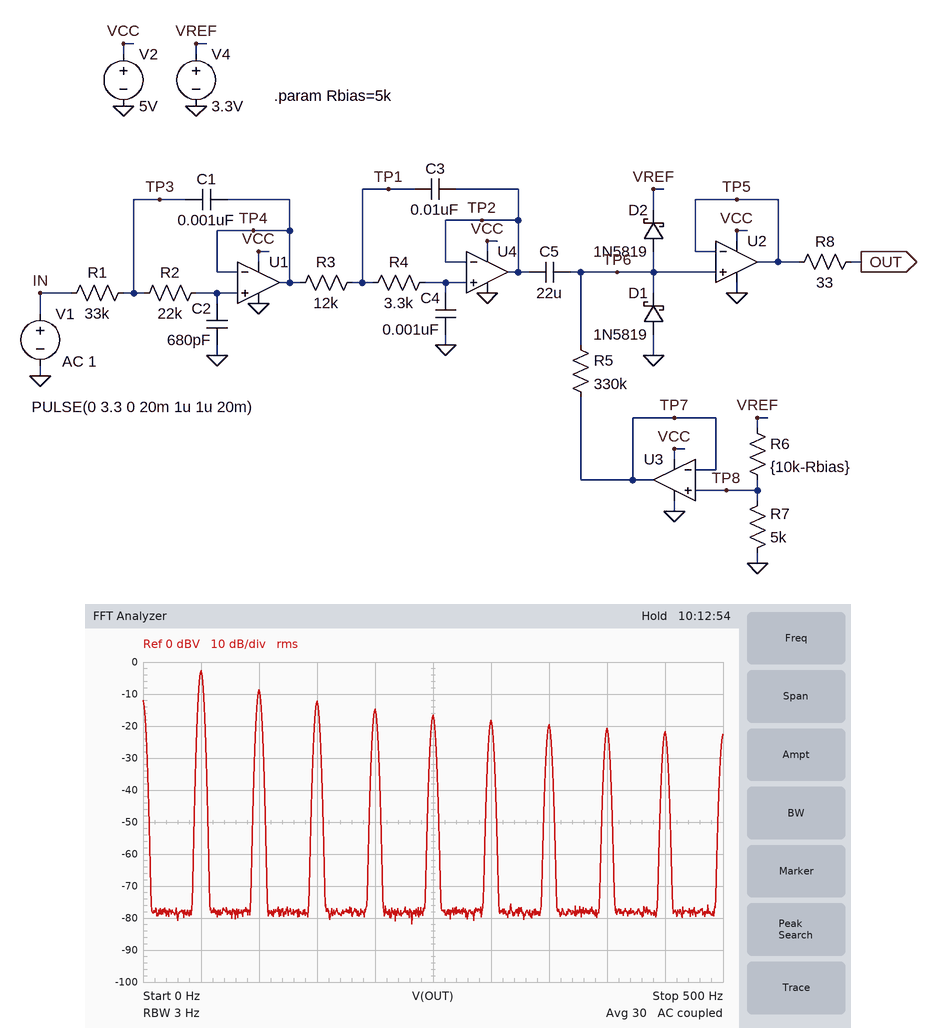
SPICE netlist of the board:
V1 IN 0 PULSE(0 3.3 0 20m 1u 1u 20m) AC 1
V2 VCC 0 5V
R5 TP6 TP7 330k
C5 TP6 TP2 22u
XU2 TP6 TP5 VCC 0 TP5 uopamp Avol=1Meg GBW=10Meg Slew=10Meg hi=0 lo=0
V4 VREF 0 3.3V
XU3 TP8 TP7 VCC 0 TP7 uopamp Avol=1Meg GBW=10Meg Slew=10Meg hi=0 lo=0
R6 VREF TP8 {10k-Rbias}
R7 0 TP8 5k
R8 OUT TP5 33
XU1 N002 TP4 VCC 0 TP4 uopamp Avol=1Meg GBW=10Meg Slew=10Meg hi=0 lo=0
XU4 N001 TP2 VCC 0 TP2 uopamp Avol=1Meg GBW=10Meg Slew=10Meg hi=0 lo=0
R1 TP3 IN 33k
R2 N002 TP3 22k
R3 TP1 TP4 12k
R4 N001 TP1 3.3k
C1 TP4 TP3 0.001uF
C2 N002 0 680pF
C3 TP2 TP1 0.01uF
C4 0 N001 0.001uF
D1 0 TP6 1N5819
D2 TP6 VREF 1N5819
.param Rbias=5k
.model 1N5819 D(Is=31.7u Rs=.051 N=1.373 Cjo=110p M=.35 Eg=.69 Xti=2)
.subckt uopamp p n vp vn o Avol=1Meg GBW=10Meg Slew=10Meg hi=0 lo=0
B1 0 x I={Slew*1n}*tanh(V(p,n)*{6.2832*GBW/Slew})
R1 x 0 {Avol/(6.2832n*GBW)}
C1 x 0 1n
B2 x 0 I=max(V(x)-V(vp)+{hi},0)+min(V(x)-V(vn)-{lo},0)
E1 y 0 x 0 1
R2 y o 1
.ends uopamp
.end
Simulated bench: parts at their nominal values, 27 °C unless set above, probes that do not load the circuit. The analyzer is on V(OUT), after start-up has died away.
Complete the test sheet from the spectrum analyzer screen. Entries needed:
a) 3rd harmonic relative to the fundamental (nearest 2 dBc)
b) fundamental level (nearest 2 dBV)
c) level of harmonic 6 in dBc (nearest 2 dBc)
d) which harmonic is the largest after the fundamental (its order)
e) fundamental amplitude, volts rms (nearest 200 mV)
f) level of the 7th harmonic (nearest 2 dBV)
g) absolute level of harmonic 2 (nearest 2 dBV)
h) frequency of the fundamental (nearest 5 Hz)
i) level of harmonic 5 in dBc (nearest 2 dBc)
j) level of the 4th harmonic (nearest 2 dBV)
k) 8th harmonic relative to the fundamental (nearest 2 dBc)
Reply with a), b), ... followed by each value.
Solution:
a) -10 dBc
b) -2 dBV
c) -16 dBc
d) 2
e) 800 mV
f) -20 dBV
g) -8 dBV
h) 50 Hz
i) -14 dBc
j) -14 dBV
k) -18 dBc
